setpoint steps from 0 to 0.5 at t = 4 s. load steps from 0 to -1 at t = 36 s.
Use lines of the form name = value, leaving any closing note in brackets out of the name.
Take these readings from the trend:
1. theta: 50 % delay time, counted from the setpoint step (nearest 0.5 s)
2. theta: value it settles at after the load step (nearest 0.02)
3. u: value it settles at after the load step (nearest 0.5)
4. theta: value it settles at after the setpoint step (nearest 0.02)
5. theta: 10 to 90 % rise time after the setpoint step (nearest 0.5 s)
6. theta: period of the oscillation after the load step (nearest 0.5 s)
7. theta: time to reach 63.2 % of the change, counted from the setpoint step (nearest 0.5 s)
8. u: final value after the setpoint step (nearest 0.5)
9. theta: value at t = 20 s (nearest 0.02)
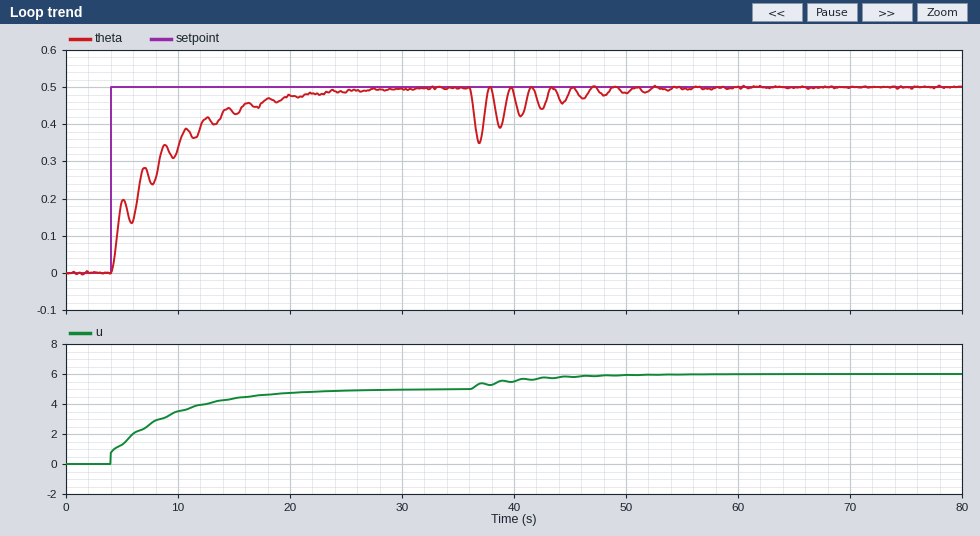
theta: 50 % delay time, counted from the setpoint step = 2.5 s
theta: value it settles at after the load step = 0.50
u: value it settles at after the load step = 6.0
theta: value it settles at after the setpoint step = 0.50
theta: 10 to 90 % rise time after the setpoint step = 11.5 s
theta: period of the oscillation after the load step = 2.0 s
theta: time to reach 63.2 % of the change, counted from the setpoint step = 4.5 s
u: final value after the setpoint step = 5.0
theta: value at t = 20 s = 0.48
